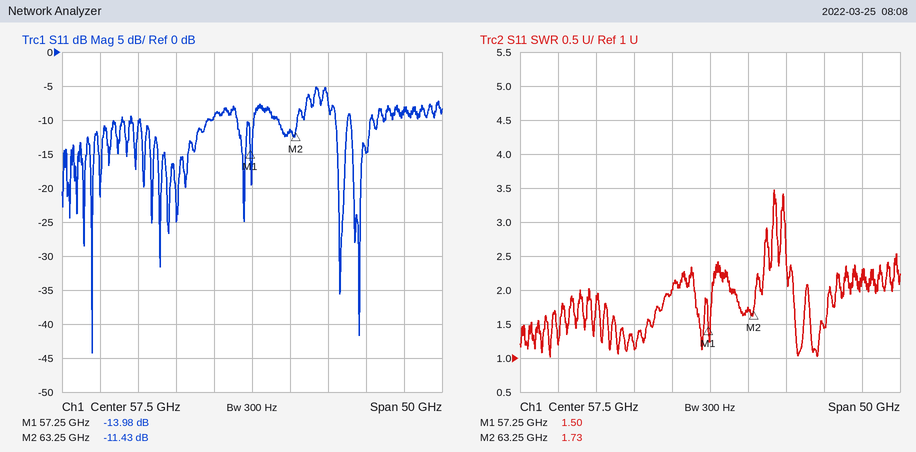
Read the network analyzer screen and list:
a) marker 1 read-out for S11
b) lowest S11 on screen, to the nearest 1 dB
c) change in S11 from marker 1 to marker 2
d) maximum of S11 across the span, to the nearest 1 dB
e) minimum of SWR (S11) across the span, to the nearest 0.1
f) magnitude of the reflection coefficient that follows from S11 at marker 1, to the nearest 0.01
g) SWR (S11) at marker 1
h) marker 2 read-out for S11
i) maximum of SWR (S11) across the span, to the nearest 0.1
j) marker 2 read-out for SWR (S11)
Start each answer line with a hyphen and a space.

- -13.98 dB
- -44 dB
- 2.55 dB
- -5 dB
- 1.0
- 0.20
- 1.50
- -11.43 dB
- 3.5
- 1.73
